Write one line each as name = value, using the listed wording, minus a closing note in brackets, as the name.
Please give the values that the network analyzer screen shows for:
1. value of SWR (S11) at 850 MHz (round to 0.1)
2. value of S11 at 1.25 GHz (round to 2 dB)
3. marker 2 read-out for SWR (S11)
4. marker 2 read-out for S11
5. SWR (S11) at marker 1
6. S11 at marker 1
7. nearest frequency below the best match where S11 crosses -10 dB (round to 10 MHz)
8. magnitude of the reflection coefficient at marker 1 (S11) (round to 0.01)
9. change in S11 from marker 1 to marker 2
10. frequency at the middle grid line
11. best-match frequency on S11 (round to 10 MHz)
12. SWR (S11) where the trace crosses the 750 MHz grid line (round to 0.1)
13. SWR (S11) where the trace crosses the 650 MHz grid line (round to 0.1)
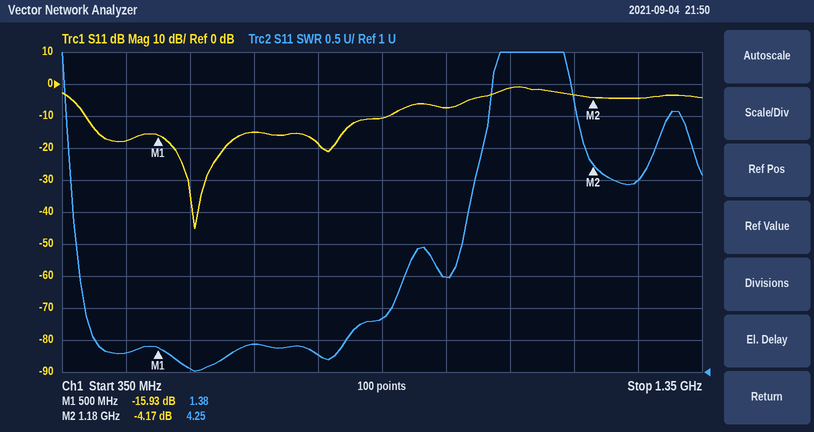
value of SWR (S11) at 850 MHz = 1.8
value of S11 at 1.25 GHz = -4 dB
marker 2 read-out for SWR = 4.25
marker 2 read-out for S11 = -4.17 dB
SWR (S11) at marker 1 = 1.38
S11 at marker 1 = -15.93 dB
nearest frequency below the best match where S11 crosses -10 dB = 390 MHz
magnitude of the reflection coefficient at marker 1 (S11) = 0.16
change in S11 from marker 1 to marker 2 = 11.76 dB
frequency at the middle grid line = 850 MHz
best-match frequency on S11 = 560 MHz
SWR (S11) where the trace crosses the 750 MHz grid line = 1.3
SWR (S11) where the trace crosses the 650 MHz grid line = 1.4
